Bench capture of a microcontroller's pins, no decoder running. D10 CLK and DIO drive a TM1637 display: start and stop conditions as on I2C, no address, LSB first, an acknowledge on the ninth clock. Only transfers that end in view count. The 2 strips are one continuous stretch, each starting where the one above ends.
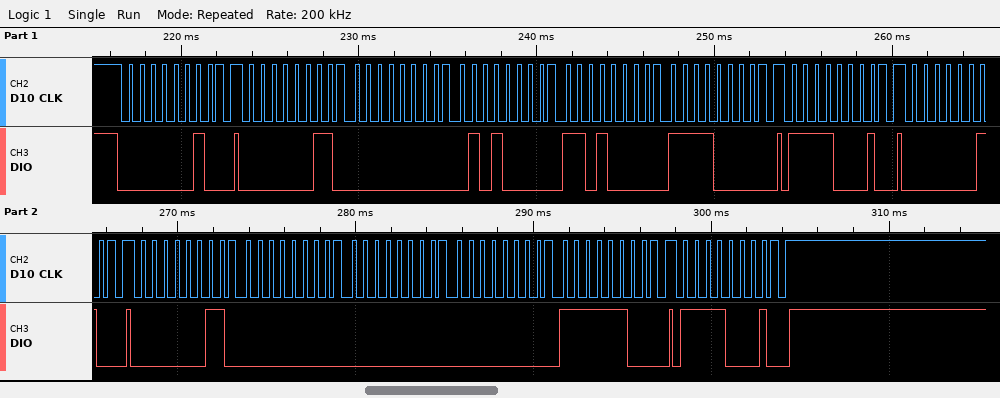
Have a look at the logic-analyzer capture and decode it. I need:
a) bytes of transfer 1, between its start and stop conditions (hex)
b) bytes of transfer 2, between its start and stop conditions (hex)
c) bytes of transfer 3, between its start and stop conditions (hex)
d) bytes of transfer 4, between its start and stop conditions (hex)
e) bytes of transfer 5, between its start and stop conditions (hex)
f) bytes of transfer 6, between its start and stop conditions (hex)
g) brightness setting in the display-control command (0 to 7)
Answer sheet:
40
C0 00 0A 0B 0F
8F
40
C0 00 00 00 3F
8F
7
